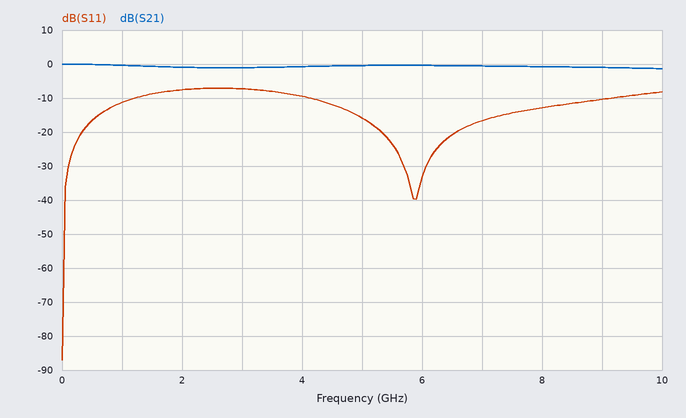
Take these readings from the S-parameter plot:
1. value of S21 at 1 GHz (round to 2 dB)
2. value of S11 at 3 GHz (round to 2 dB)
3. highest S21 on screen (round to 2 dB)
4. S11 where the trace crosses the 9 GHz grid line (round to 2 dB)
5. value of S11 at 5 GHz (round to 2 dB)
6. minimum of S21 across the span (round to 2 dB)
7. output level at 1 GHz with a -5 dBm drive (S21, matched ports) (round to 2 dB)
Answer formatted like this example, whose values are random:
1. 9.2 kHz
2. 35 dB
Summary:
1. 0 dB
2. -8 dB
3. 0 dB
4. -10 dB
5. -16 dB
6. -2 dB
7. -6 dBm
